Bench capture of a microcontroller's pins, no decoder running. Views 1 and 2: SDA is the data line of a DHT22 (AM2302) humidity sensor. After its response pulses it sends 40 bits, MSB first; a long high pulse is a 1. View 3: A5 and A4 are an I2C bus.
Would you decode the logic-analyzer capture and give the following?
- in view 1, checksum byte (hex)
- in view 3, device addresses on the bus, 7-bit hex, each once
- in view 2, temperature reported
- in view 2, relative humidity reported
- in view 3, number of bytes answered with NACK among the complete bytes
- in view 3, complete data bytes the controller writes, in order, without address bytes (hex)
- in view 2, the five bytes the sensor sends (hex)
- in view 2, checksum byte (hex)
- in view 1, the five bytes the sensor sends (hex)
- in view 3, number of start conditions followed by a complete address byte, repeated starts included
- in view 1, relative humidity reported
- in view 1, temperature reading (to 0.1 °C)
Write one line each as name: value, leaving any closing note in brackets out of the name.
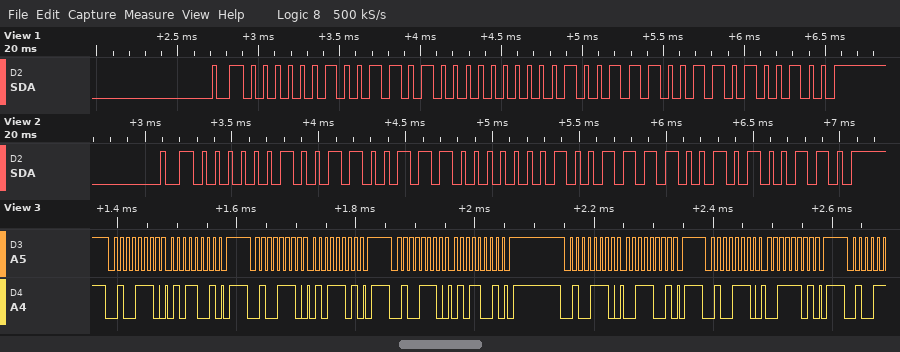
in view 1, checksum byte: 0xA4
in view 3, device addresses on the bus, 7-bit hex, each once: 0x27
in view 2, temperature reported: 31.6 °C
in view 2, relative humidity reported: 61.5 %
in view 3, number of bytes answered with NACK among the complete bytes: 0
in view 3, complete data bytes the controller writes, in order, without address bytes: 59 5D 59 39 3D
in view 2, the five bytes the sensor sends: 02 67 01 3C A6
in view 2, checksum byte: 0xA6
in view 1, the five bytes the sensor sends: 02 68 01 39 A4
in view 3, number of start conditions followed by a complete address byte, repeated starts included: 5
in view 1, relative humidity reported: 61.6 %
in view 1, temperature reading: 31.3 °C
